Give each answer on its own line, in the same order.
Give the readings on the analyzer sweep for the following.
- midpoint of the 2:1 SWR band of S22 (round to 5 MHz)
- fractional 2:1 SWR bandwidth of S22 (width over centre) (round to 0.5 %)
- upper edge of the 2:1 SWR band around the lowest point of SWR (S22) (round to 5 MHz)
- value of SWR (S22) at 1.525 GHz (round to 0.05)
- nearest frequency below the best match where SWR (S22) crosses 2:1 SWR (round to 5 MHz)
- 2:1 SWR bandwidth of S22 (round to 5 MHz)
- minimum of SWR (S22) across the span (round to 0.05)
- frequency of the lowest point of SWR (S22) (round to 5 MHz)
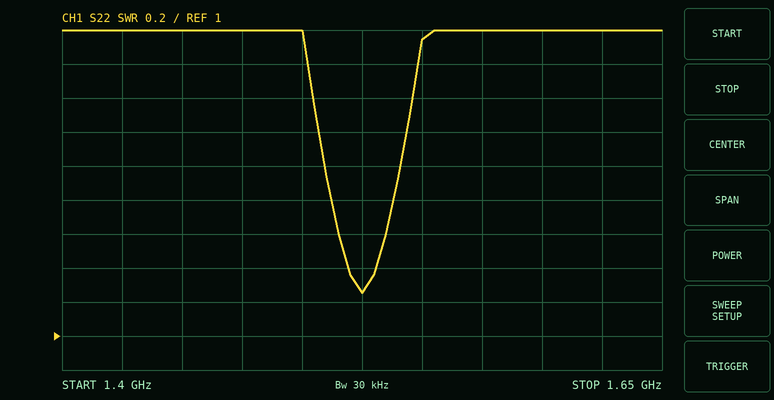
1.525 GHz
2.0 %
1.540 GHz
1.25
1.510 GHz
30 MHz
1.25
1.525 GHz
